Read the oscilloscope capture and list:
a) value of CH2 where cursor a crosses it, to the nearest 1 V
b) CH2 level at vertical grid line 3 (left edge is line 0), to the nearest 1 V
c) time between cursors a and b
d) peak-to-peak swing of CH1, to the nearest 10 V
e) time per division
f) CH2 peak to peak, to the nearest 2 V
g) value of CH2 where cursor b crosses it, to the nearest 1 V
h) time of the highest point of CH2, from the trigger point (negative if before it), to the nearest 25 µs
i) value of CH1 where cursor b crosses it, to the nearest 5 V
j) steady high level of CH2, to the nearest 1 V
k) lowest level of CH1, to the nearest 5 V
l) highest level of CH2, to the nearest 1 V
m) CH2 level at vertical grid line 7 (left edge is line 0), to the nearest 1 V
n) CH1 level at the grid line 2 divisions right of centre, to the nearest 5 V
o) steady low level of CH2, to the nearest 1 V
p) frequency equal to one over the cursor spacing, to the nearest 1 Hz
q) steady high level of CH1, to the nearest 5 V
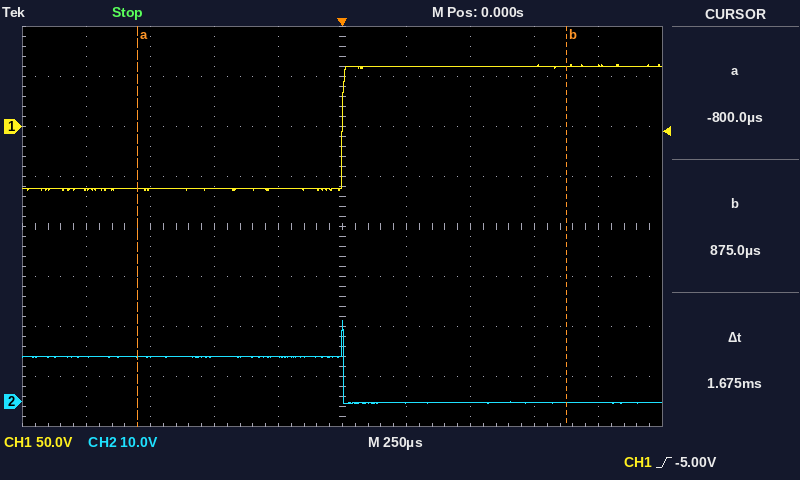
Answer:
9 V
9 V
1.675 ms
130 V
250 µs
16 V
0 V
0 µs
60 V
9 V
-65 V
16 V
0 V
60 V
0 V
597 Hz
60 V
